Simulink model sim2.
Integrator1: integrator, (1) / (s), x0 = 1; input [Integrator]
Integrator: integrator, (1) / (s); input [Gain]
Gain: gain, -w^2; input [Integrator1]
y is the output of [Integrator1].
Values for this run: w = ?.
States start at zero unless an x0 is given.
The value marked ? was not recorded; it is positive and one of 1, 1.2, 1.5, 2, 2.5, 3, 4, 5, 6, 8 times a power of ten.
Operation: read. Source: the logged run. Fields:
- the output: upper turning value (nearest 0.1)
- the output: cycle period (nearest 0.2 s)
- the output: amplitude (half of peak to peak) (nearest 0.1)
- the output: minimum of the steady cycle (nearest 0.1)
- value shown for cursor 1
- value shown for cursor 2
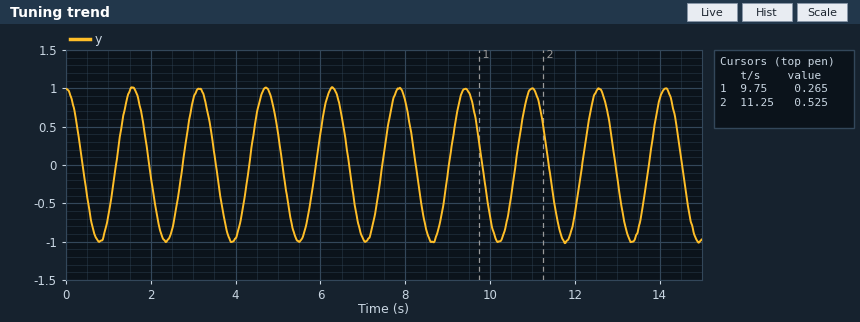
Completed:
1.0
1.6 s
1.0
-1.0
0.265
0.525
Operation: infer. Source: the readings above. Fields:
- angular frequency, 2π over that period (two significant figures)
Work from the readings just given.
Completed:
3.9 rad/s
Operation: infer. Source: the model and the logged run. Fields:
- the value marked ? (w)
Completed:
4
